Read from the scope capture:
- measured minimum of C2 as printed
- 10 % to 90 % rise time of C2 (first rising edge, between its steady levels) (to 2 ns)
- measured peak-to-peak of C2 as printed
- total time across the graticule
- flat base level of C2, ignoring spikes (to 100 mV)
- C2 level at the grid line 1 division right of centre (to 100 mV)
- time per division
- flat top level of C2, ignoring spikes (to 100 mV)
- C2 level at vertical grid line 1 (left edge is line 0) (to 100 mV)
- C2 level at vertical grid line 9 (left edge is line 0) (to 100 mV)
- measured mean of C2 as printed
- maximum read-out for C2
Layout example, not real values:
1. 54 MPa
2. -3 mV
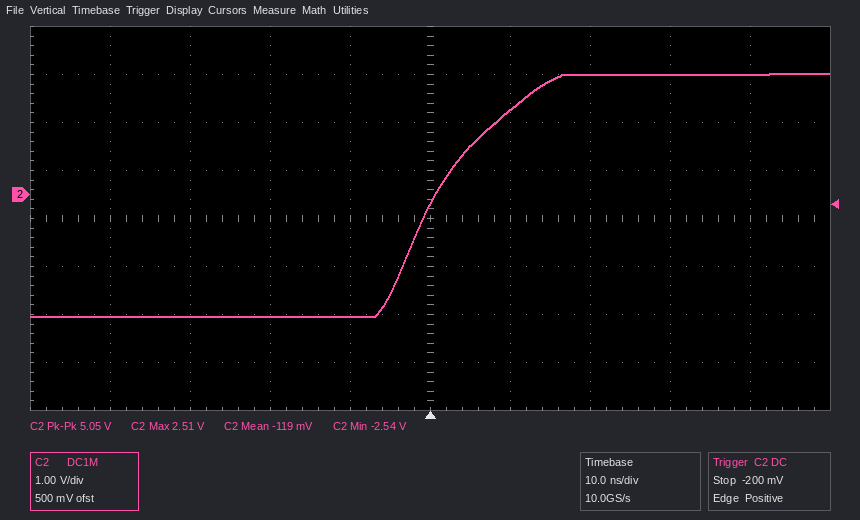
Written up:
1. -2.54 V
2. 16 ns
3. 5.05 V
4. 100 ns
5. -2.5 V
6. 1.8 V
7. 10 ns
8. 2.5 V
9. -2.5 V
10. 2.5 V
11. -119 mV
12. 2.51 V
